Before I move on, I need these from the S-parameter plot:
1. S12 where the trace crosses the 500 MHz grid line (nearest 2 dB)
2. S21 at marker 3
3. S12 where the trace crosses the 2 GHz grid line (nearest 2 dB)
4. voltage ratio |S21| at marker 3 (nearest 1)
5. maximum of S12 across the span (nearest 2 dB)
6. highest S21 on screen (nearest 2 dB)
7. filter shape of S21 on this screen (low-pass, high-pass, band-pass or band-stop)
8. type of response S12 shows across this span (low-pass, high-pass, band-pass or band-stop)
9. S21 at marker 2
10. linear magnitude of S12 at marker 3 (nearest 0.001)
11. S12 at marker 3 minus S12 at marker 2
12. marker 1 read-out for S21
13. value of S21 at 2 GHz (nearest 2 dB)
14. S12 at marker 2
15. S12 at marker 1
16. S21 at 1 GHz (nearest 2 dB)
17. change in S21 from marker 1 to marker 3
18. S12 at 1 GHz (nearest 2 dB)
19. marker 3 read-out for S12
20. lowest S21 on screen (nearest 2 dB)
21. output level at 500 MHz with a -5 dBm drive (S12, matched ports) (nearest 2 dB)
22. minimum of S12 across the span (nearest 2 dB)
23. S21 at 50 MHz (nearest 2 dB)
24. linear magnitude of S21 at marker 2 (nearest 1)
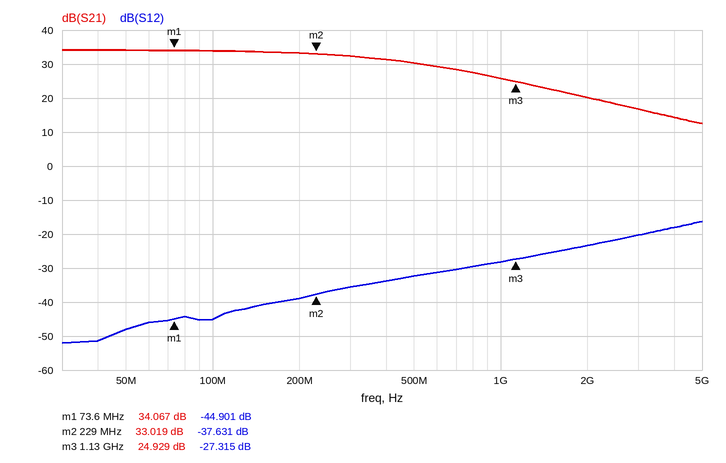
-32 dB
24.929 dB
-24 dB
18
-16 dB
34 dB
low-pass
high-pass
33.019 dB
0.043
10.316 dB
34.067 dB
20 dB
-37.631 dB
-44.901 dB
26 dB
-9.138 dB
-28 dB
-27.315 dB
12 dB
-38 dBm
-52 dB
34 dB
45
